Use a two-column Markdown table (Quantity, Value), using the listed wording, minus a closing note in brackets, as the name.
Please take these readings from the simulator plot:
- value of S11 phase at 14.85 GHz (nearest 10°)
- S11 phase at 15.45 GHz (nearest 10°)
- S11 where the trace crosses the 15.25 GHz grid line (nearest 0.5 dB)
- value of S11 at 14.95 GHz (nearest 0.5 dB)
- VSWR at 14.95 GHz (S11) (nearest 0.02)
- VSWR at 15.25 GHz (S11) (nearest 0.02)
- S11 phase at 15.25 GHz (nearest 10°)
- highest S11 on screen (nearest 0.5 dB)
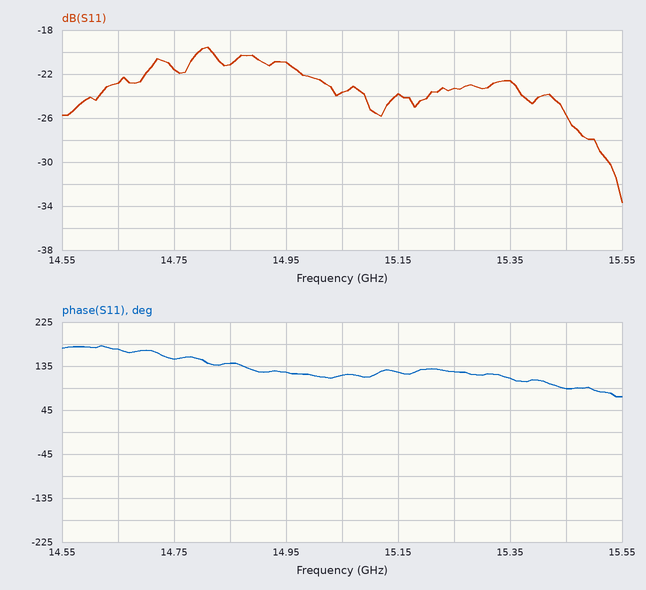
| Quantity | Value |
|---|---|
| value of S11 phase at 14.85 GHz | 140° |
| S11 phase at 15.45 GHz | 90° |
| S11 where the trace crosses the 15.25 GHz grid line | -23.5 dB |
| value of S11 at 14.95 GHz | -21.0 dB |
| VSWR at 14.95 GHz (S11) | 1.20 |
| VSWR at 15.25 GHz (S11) | 1.14 |
| S11 phase at 15.25 GHz | 120° |
| highest S11 on screen | -19.5 dB |
